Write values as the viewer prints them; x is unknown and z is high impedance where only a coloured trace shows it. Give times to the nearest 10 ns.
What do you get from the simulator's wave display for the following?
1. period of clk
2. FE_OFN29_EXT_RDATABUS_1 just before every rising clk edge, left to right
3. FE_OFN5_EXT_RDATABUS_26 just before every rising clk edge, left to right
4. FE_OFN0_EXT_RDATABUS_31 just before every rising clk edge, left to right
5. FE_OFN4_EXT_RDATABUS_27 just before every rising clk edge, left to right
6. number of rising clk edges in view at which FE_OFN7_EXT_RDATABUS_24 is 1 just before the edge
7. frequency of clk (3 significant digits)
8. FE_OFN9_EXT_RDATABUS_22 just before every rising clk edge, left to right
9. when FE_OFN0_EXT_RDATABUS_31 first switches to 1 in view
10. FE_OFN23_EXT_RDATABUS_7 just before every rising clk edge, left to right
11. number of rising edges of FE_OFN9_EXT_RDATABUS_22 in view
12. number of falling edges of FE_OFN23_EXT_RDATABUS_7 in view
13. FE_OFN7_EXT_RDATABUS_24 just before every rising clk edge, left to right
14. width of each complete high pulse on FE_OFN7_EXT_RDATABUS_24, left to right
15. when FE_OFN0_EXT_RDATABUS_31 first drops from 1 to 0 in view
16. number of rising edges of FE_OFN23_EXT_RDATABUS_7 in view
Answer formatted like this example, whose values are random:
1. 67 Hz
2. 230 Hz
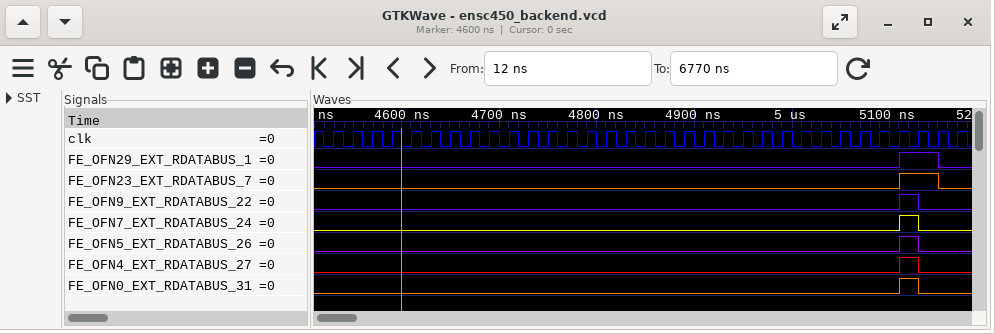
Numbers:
1. 20 ns
2. 0 0 0 0 0 0 0 0 0 0 0 0 0 0 0 0 0 0 0 0 0 0 0 0 0 0 0 0 0 0 1 1 0
3. 0 0 0 0 0 0 0 0 0 0 0 0 0 0 0 0 0 0 0 0 0 0 0 0 0 0 0 0 0 0 1 0 0
4. 0 0 0 0 0 0 0 0 0 0 0 0 0 0 0 0 0 0 0 0 0 0 0 0 0 0 0 0 0 0 1 0 0
5. 0 0 0 0 0 0 0 0 0 0 0 0 0 0 0 0 0 0 0 0 0 0 0 0 0 0 0 0 0 0 1 0 0
6. 1
7. 50.0 MHz
8. 0 0 0 0 0 0 0 0 0 0 0 0 0 0 0 0 0 0 0 0 0 0 0 0 0 0 0 0 0 0 1 0 0
9. 5110 ns
10. 0 0 0 0 0 0 0 0 0 0 0 0 0 0 0 0 0 0 0 0 0 0 0 0 0 0 0 0 0 0 1 1 0
11. 1
12. 1
13. 0 0 0 0 0 0 0 0 0 0 0 0 0 0 0 0 0 0 0 0 0 0 0 0 0 0 0 0 0 0 1 0 0
14. 20 ns
15. 5130 ns
16. 1
